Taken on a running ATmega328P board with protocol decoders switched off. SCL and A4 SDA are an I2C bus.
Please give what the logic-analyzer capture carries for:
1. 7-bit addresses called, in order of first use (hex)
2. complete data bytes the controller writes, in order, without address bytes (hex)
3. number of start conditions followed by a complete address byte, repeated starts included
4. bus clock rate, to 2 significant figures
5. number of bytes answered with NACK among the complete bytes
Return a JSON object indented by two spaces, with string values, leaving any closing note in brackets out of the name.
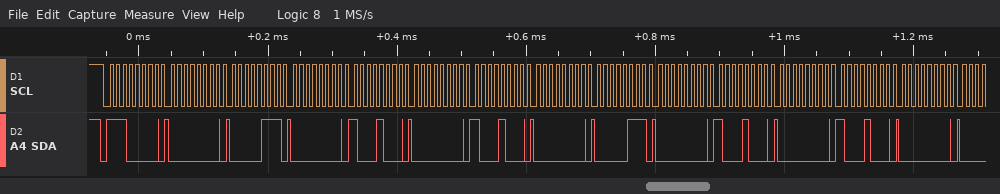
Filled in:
{
  "7-bit addresses called, in order of first use": "0x70",
  "complete data bytes the controller writes, in order, without address bytes": "00 07 00 88 00 88 00 07 00 88 00 88 00",
  "number of start conditions followed by a complete address byte, repeated starts included": "1",
  "bus clock rate, to 2 significant figures": "100 kHz",
  "number of bytes answered with NACK among the complete bytes": "0"
}
